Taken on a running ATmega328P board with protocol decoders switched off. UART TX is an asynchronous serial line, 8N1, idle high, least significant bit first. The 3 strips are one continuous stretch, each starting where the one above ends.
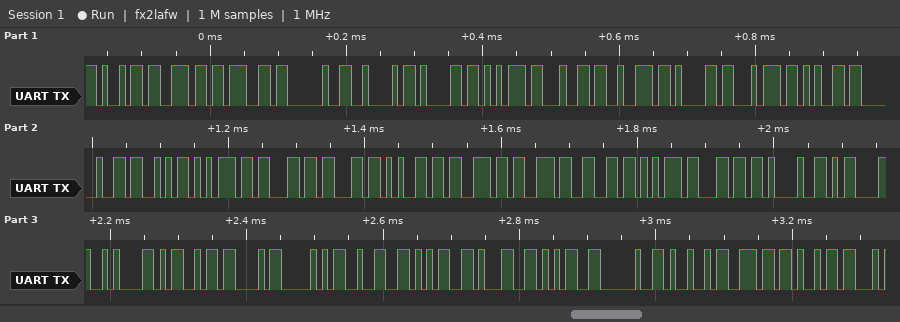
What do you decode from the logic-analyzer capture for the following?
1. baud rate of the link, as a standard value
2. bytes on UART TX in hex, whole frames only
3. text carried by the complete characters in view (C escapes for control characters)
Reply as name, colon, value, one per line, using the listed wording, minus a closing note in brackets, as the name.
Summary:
baud rate of the link, as a standard value: 115200 baud
bytes on UART TX in hex, whole frames only: 69 6E 67 20 42 61 75 64 72 61 74 65 20 53 75 63 63 65 73 73 66 75 6C 21 0D 0A 4D 43 50 32 35 31 35 20 49 6E 69
text carried by the complete characters in view: "ing Baudrate Successful!\r\nMCP2515 Ini"
